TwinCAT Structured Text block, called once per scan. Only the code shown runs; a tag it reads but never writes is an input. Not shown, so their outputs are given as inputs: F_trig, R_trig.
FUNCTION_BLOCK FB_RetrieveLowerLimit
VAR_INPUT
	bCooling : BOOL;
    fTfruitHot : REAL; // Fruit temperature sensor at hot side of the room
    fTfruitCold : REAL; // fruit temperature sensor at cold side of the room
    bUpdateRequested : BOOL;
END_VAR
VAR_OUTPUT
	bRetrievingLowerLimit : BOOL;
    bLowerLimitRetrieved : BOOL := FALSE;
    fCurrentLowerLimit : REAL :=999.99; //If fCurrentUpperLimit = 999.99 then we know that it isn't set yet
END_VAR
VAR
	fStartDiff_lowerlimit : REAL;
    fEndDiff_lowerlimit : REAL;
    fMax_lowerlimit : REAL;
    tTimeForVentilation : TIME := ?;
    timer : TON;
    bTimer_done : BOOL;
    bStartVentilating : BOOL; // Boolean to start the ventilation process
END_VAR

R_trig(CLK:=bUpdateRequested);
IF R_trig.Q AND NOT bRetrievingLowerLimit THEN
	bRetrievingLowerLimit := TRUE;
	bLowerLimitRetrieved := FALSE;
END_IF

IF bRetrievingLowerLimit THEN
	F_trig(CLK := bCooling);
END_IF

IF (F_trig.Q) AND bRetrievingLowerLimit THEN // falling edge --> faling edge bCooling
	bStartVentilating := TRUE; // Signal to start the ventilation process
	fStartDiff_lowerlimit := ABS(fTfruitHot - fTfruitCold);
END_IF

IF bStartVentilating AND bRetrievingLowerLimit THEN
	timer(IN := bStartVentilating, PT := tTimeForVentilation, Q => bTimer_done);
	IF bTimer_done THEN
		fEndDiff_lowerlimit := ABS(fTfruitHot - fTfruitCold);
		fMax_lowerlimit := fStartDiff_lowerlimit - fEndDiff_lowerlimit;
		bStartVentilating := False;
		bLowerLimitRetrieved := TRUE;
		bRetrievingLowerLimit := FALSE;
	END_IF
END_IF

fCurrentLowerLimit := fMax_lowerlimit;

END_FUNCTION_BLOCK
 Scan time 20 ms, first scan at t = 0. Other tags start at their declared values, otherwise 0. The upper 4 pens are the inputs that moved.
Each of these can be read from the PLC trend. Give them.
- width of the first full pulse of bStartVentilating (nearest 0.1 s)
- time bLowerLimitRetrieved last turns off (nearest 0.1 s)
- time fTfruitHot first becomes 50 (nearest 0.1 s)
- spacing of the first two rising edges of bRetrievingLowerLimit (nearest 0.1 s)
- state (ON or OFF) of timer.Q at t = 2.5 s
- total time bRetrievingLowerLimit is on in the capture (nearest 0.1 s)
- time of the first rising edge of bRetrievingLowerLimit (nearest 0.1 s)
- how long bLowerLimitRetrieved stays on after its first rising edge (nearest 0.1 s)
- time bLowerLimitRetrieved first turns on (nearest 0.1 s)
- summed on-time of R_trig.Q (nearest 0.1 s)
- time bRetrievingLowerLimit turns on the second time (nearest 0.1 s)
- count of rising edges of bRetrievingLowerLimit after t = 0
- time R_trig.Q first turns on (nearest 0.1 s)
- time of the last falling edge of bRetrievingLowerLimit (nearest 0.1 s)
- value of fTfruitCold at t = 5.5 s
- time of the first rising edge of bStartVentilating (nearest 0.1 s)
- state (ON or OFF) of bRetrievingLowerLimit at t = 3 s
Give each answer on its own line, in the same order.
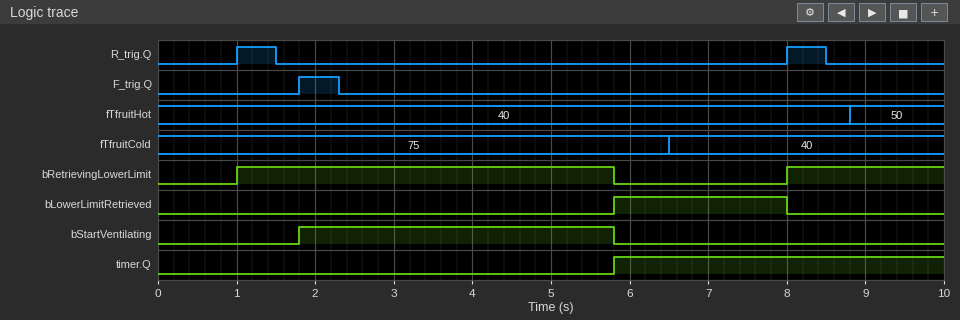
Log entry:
4.0 s
8.0 s
8.8 s
7.0 s
OFF
6.8 s
1.0 s
2.2 s
5.8 s
1.0 s
8.0 s
2
1.0 s
5.8 s
75
1.8 s
ON
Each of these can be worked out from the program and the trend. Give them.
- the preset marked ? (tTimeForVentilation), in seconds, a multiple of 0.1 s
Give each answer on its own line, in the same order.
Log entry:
4.0 s
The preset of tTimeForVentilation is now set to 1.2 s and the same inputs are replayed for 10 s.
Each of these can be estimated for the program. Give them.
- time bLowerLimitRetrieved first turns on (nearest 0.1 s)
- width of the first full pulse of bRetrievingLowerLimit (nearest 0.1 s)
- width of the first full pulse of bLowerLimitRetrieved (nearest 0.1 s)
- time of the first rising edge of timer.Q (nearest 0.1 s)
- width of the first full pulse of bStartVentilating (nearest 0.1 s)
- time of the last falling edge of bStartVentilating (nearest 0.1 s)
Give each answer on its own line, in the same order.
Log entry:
3.0 s
2.0 s
5.0 s
3.0 s
1.2 s
3.0 s
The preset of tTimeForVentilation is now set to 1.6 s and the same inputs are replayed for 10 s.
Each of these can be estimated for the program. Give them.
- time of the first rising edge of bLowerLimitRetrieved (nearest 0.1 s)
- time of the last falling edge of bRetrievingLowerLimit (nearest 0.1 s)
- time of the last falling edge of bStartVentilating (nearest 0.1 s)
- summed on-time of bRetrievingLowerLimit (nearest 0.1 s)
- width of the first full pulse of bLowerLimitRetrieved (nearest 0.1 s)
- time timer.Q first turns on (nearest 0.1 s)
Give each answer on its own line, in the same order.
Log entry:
3.4 s
3.4 s
3.4 s
4.4 s
4.6 s
3.4 s
